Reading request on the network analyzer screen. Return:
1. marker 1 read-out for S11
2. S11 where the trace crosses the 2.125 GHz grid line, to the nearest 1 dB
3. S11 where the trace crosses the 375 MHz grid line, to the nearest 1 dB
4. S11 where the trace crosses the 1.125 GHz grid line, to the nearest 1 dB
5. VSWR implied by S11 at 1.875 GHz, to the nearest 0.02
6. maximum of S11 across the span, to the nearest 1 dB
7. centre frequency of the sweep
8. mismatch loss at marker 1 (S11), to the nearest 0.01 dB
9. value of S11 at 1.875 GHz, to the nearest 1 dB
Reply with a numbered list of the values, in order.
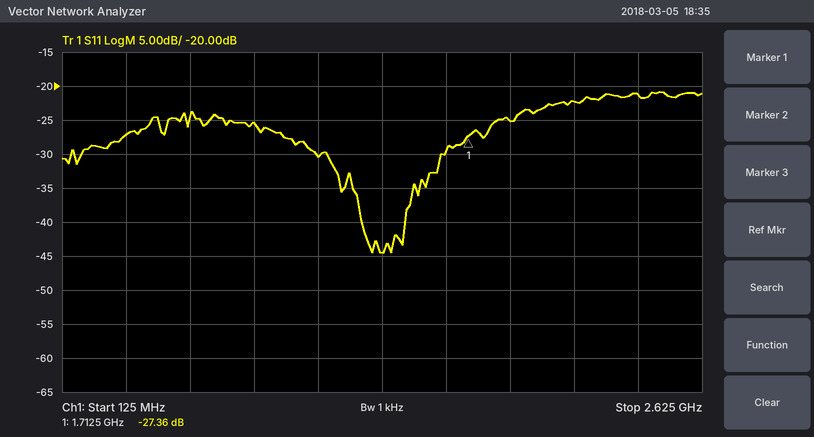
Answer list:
1. -27.36 dB
2. -22 dB
3. -27 dB
4. -30 dB
5. 1.12
6. -21 dB
7. 1.375 GHz
8. 0.01 dB
9. -25 dB
